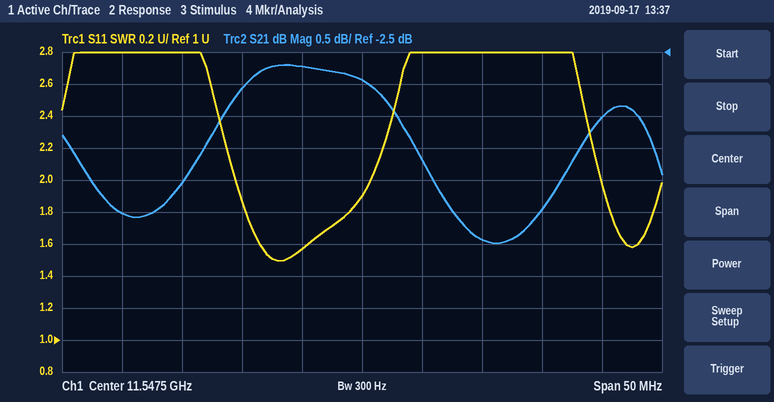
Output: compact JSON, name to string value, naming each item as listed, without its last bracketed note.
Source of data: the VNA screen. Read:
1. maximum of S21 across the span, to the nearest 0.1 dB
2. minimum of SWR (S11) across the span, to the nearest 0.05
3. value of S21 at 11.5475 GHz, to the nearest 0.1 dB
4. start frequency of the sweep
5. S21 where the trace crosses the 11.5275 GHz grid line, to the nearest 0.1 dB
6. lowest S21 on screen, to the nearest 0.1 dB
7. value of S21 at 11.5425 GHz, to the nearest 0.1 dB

{"maximum of S21 across the span, to the nearest 0.1 dB": "-2.7 dB", "minimum of SWR (S11) across the span, to the nearest 0.05": "1.50", "value of S21 at 11.5475 GHz, to the nearest 0.1 dB": "-2.9 dB", "start frequency of the sweep": "11.5225 GHz", "S21 where the trace crosses the 11.5275 GHz grid line, to the nearest 0.1 dB": "-5.0 dB", "lowest S21 on screen, to the nearest 0.1 dB": "-5.5 dB", "value of S21 at 11.5425 GHz, to the nearest 0.1 dB": "-2.7 dB"}
